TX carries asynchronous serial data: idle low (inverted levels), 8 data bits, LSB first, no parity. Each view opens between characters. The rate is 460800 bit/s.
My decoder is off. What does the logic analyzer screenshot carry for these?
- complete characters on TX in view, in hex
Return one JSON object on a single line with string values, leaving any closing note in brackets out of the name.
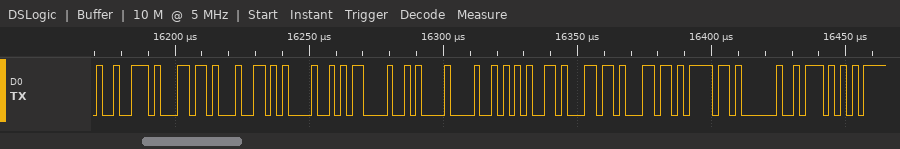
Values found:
{"complete characters on TX in view, in hex": "1B, 27, 37, BD, E5, EB, 6F, 35, 27, 27, 21, BF, 51"}
